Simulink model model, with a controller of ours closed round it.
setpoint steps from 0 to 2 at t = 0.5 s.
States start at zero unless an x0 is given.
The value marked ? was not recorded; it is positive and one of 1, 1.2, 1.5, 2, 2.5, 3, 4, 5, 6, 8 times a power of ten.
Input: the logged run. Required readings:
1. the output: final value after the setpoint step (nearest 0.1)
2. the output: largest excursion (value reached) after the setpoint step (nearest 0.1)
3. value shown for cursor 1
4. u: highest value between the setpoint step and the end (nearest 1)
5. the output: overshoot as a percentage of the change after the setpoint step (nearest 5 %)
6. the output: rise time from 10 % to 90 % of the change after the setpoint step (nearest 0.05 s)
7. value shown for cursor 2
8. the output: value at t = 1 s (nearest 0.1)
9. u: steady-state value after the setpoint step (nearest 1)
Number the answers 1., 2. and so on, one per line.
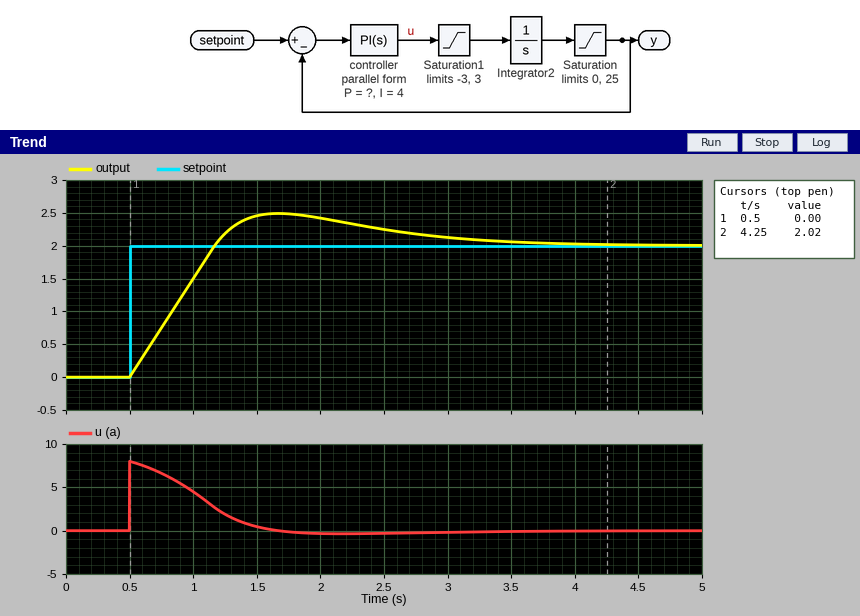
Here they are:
1. 2.0
2. 2.5
3. 0.00
4. 8
5. 25 %
6. 0.55 s
7. 2.02
8. 1.5
9. 0
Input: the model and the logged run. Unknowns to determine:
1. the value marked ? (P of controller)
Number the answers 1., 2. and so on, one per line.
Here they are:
1. 4
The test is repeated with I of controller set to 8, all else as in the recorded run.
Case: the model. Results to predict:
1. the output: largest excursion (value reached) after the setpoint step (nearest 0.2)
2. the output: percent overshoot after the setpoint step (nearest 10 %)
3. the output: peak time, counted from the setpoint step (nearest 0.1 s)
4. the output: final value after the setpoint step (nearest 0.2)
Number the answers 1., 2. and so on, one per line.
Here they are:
1. 2.8
2. 40 %
3. 1.1 s
4. 2.0
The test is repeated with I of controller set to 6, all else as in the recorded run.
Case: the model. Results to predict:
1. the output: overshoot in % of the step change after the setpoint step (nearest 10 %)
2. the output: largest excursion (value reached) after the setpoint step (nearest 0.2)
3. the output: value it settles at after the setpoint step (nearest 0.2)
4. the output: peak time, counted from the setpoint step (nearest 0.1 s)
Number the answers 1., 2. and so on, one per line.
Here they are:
1. 30 %
2. 2.6
3. 2.0
4. 1.1 s
